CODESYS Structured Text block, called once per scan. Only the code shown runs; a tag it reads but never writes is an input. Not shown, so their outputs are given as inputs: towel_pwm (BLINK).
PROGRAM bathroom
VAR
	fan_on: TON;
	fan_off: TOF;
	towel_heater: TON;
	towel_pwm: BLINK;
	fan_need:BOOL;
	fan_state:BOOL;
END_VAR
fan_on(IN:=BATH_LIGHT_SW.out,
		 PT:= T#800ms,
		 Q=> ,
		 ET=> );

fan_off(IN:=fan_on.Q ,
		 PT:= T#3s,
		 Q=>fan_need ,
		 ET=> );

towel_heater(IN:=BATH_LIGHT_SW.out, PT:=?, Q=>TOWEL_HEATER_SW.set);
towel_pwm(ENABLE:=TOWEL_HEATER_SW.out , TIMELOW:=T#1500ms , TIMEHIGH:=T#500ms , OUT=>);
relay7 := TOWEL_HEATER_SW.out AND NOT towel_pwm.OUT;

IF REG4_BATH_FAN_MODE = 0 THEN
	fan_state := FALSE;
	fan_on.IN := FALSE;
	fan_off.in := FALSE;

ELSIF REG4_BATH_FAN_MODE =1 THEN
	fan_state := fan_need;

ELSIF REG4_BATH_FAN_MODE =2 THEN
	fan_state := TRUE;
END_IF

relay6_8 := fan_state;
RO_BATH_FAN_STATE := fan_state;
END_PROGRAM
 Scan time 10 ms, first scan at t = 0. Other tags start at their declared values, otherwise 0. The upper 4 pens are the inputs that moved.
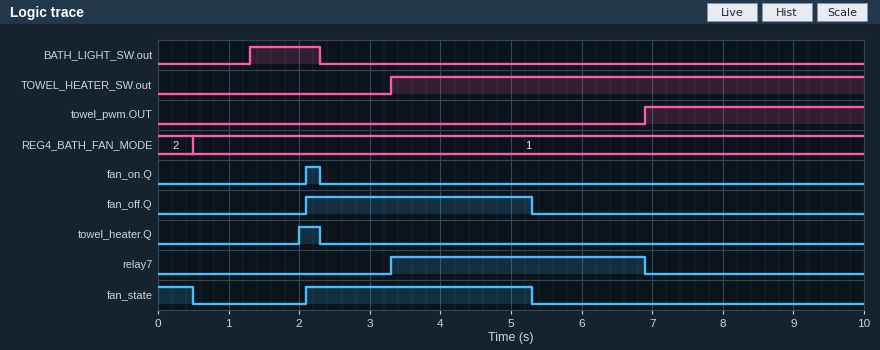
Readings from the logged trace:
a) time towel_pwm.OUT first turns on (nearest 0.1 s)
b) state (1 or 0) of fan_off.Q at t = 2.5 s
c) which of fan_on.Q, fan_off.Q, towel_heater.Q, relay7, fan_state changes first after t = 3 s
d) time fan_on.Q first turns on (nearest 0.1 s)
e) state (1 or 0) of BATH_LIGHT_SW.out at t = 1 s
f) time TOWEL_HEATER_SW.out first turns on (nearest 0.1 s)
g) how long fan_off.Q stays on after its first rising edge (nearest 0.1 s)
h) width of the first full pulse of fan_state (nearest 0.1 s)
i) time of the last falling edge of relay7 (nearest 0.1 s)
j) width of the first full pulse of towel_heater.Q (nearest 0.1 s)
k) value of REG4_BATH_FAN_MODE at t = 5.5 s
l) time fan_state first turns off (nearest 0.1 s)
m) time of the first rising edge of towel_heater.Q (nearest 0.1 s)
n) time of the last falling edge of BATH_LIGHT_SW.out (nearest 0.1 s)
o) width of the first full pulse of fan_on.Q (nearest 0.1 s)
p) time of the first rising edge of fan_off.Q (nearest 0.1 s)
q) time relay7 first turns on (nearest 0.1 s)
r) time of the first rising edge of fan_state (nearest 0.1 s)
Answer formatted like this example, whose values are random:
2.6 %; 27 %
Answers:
6.9 s; 1; relay7; 2.1 s; 0; 3.3 s; 3.2 s; 3.2 s; 6.9 s; 0.3 s; 1; 0.5 s; 2.0 s; 2.3 s; 0.2 s; 2.1 s; 3.3 s; 2.1 s
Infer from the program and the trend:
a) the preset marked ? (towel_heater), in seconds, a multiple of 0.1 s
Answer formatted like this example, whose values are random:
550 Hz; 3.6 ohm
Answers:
0.7 s
